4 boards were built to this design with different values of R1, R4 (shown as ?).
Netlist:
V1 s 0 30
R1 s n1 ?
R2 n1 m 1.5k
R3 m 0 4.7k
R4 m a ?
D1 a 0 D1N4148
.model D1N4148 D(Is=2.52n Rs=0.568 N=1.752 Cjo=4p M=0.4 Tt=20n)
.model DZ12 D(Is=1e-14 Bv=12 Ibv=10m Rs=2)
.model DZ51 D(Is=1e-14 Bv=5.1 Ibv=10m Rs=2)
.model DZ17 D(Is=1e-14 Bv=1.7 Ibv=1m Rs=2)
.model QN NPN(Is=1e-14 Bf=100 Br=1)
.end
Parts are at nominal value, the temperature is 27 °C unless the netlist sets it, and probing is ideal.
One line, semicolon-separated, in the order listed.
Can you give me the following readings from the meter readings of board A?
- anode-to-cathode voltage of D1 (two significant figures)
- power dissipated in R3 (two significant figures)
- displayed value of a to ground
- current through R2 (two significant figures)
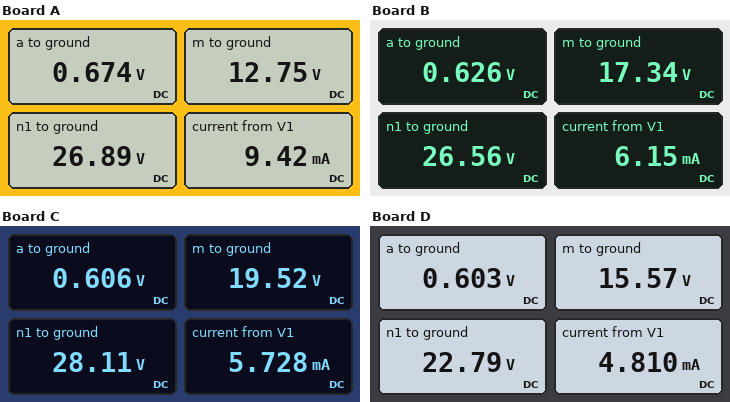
670 mV; 35 mW; 0.674 V; 9.4 mA
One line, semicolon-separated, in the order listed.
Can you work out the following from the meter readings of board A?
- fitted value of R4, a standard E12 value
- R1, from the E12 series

1.8 kΩ; 330 Ω
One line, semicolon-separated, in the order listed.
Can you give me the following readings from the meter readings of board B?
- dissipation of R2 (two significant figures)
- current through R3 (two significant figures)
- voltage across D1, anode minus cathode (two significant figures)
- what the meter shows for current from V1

57 mW; 3.7 mA; 630 mV; 6.15 mA
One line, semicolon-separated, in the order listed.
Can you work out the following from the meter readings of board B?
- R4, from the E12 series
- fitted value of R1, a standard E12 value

6.8 kΩ; 560 Ω
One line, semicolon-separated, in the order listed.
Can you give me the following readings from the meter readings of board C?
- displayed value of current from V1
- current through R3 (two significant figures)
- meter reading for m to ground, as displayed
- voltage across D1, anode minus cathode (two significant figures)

5.728 mA; 4.2 mA; 19.52 V; 610 mV
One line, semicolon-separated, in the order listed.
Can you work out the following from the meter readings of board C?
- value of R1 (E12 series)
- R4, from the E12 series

330 Ω; 12 kΩ
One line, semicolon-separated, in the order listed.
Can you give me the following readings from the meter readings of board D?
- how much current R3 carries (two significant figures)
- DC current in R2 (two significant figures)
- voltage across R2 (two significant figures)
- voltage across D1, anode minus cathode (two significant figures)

3.3 mA; 4.8 mA; 7.2 V; 600 mV
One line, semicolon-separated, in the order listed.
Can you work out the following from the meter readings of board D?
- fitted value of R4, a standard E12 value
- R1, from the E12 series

10 kΩ; 1.5 kΩ
